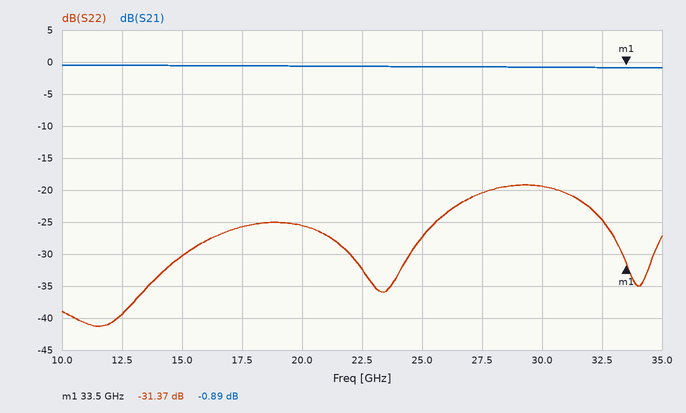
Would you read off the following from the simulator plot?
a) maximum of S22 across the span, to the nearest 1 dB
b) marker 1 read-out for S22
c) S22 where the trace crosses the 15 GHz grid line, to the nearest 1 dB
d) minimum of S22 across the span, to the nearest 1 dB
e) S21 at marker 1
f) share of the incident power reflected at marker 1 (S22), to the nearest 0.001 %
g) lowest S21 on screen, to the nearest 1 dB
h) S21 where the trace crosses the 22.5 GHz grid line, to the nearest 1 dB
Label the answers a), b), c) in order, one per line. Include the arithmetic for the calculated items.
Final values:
a) -19 dB
b) -31.37 dB
c) -30 dB
d) -41 dB
e) -0.89 dB
f) 10^(-31.37/10) ≈ 0.073 %
g) -1 dB
h) -1 dB
